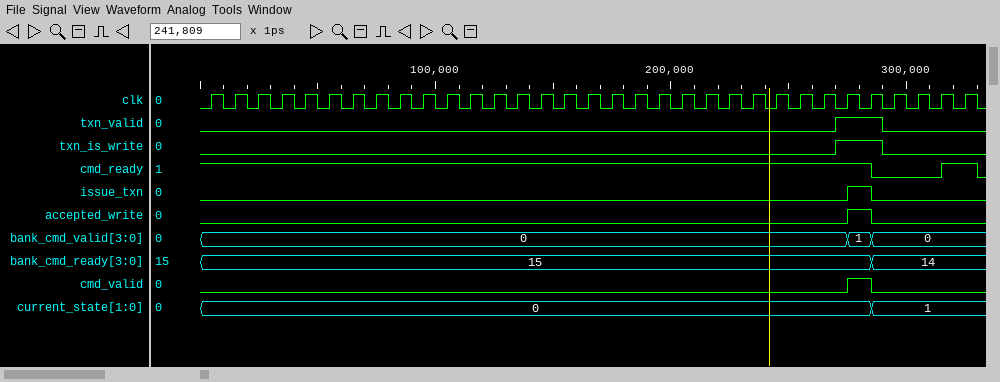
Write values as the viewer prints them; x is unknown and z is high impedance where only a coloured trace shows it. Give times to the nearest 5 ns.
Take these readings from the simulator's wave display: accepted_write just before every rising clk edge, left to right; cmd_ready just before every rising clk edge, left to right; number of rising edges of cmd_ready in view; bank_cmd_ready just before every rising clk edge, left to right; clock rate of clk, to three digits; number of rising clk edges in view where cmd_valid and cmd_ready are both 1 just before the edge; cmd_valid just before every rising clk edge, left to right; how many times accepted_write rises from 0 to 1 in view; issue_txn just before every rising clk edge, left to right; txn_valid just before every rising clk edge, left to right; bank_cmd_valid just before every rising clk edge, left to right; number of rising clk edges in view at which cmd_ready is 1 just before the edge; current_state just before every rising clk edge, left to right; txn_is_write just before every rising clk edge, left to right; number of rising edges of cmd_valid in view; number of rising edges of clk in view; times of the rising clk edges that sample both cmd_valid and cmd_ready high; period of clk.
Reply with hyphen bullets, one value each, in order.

- 0 0 0 0 0 0 0 0 0 0 0 0 0 0 0 0 0 0 0 0 0 0 0 0 0 0 0 0 1 0 0 0 0
- 1 1 1 1 1 1 1 1 1 1 1 1 1 1 1 1 1 1 1 1 1 1 1 1 1 1 1 1 1 0 0 0 1
- 1
- 15, 15, 15, 15, 15, 15, 15, 15, 15, 15, 15, 15, 15, 15, 15, 15, 15, 15, 15, 15, 15, 15, 15, 15, 15, 15, 15, 15, 15, 14, 14, 14, 14
- 100 MHz
- 1
- 0 0 0 0 0 0 0 0 0 0 0 0 0 0 0 0 0 0 0 0 0 0 0 0 0 0 0 0 1 0 0 0 0
- 1
- 0 0 0 0 0 0 0 0 0 0 0 0 0 0 0 0 0 0 0 0 0 0 0 0 0 0 0 0 1 0 0 0 0
- 0 0 0 0 0 0 0 0 0 0 0 0 0 0 0 0 0 0 0 0 0 0 0 0 0 0 0 1 1 0 0 0 0
- 0, 0, 0, 0, 0, 0, 0, 0, 0, 0, 0, 0, 0, 0, 0, 0, 0, 0, 0, 0, 0, 0, 0, 0, 0, 0, 0, 0, 1, 0, 0, 0, 0
- 30
- 0, 0, 0, 0, 0, 0, 0, 0, 0, 0, 0, 0, 0, 0, 0, 0, 0, 0, 0, 0, 0, 0, 0, 0, 0, 0, 0, 0, 0, 1, 1, 1, 1
- 0 0 0 0 0 0 0 0 0 0 0 0 0 0 0 0 0 0 0 0 0 0 0 0 0 0 0 1 1 0 0 0 0
- 1
- 33
- 285 ns
- 10 ns
